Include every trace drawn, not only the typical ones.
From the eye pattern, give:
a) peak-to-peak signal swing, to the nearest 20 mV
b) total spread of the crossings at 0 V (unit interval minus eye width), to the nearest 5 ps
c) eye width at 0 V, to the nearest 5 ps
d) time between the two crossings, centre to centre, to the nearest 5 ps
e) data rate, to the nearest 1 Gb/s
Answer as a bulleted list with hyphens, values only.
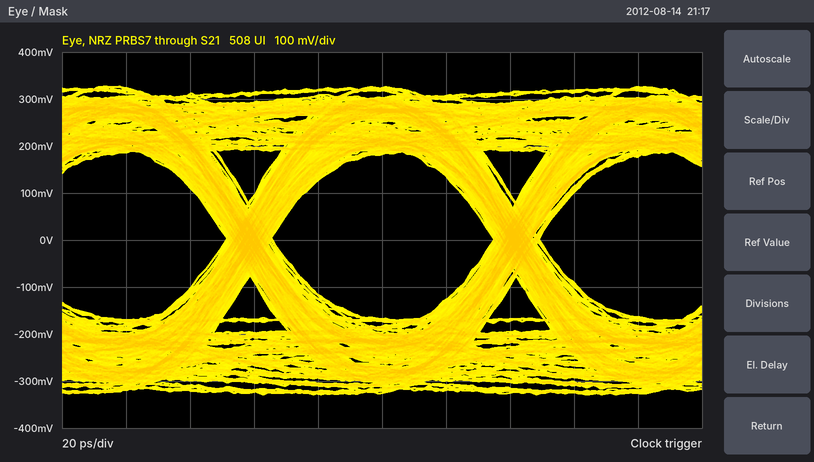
- 660 mV
- 15 ps
- 70 ps
- 85 ps
- 12 Gb/s
